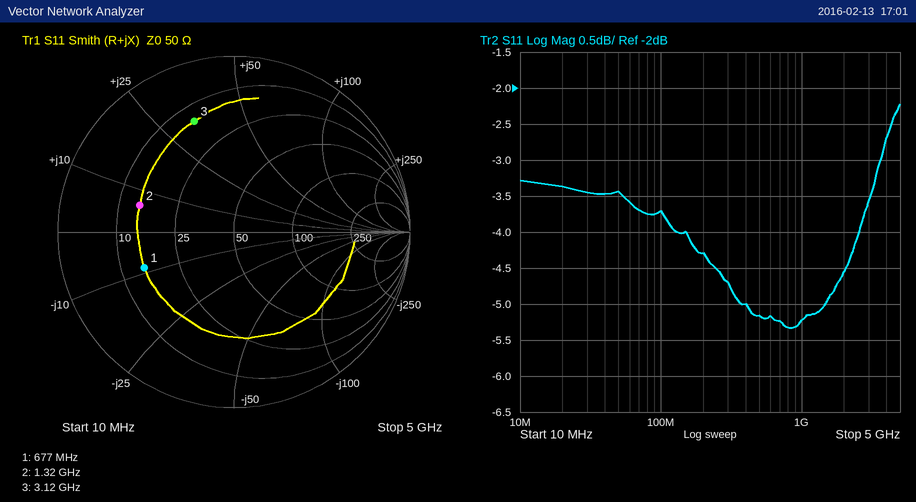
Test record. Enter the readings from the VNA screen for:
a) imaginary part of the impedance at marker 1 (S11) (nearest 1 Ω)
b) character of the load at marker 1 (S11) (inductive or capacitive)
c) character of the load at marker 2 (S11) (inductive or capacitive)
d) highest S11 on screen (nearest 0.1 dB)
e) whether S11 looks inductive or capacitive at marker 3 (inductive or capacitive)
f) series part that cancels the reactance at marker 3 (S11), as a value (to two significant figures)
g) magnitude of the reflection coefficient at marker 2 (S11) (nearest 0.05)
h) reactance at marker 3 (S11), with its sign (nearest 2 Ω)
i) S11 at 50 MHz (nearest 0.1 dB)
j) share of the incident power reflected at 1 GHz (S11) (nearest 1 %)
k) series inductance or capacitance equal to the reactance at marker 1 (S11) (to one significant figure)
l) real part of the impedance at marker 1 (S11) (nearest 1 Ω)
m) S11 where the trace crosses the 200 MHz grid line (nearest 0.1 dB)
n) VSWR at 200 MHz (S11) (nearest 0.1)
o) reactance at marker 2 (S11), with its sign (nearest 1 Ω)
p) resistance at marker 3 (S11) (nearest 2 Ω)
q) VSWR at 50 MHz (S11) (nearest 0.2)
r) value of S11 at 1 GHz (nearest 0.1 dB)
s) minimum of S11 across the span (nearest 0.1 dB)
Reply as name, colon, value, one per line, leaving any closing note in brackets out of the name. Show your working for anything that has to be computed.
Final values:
imaginary part of the impedance at marker 1 (S11): -9 Ω
character of the load at marker 1 (S11): capacitive
character of the load at marker 2 (S11): inductive
highest S11 on screen: -2.2 dB
whether S11 looks inductive or capacitive at marker 3: inductive
series part that cancels the reactance at marker 3 (S11), as a value: C = 1/(2π × 3.12 GHz × 34 Ω) ≈ 1.5 pF
magnitude of the reflection coefficient at marker 2 (S11): 0.55
reactance at marker 3 (S11), with its sign: +34 Ω
S11 at 50 MHz: -3.4 dB
share of the incident power reflected at 1 GHz (S11): 10^(-5.2/10) ≈ 30 %
series inductance or capacitance equal to the reactance at marker 1 (S11): C = 1/(2π × 677 MHz × 9 Ω) ≈ 26.1 pF, so 30 pF to one significant figure
real part of the impedance at marker 1 (S11): 15 Ω
S11 where the trace crosses the 200 MHz grid line: -4.3 dB
VSWR at 200 MHz (S11): |Γ| = 10^(-4.3/20) = 0.6095; VSWR = (1 + 0.6095)/(1 − 0.6095) ≈ 4.1
reactance at marker 2 (S11), with its sign: +6 Ω
resistance at marker 3 (S11): 14 Ω
VSWR at 50 MHz (S11): |Γ| = 10^(-3.4/20) = 0.6761; VSWR = (1 + 0.6761)/(1 − 0.6761) ≈ 5.2
value of S11 at 1 GHz: -5.2 dB
minimum of S11 across the span: -5.3 dB
